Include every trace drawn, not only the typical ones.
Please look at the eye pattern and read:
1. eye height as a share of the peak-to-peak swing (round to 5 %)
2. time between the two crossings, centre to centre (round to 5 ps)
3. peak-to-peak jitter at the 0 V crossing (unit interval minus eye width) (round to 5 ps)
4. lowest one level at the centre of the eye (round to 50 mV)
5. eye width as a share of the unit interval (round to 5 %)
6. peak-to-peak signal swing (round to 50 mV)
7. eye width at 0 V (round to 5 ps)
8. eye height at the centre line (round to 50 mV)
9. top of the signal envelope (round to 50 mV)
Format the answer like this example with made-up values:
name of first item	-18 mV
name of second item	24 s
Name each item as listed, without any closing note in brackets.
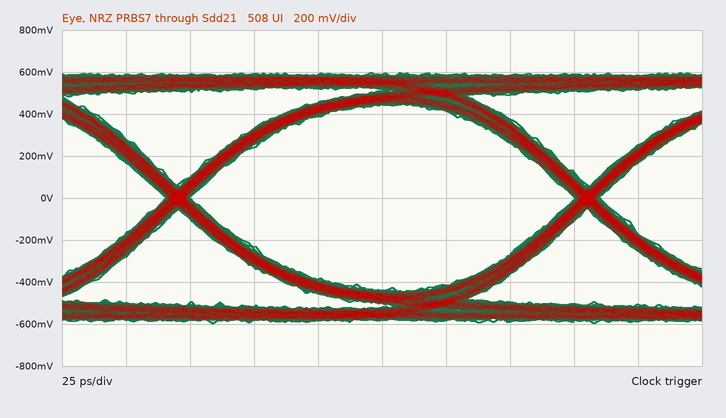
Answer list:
eye height as a share of the peak-to-peak swing	75 %
time between the two crossings, centre to centre	160 ps
peak-to-peak jitter at the 0 V crossing (unit interval minus eye width)	10 ps
lowest one level at the centre of the eye	450 mV
eye width as a share of the unit interval	95 %
peak-to-peak signal swing	1.20 V
eye width at 0 V	150 ps
eye height at the centre line	900 mV
top of the signal envelope	600 mV
